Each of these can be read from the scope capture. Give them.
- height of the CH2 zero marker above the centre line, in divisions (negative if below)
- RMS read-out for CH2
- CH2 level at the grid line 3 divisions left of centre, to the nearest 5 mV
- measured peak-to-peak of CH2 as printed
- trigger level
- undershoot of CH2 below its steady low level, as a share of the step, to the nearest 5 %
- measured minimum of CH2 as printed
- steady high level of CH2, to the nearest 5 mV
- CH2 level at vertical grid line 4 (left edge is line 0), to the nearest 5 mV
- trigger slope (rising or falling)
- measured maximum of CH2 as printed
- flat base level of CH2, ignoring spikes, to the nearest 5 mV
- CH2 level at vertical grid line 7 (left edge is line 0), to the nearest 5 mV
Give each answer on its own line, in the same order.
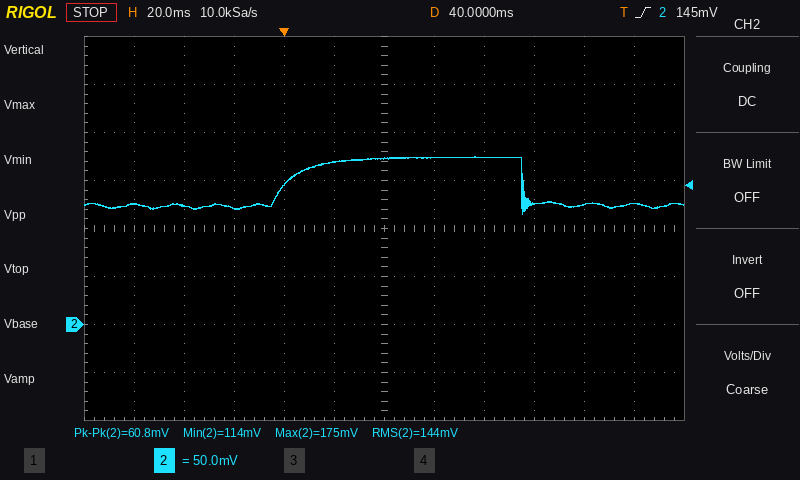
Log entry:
-2.0 div
144 mV
120 mV
60.8 mV
145 mV
20 %
114 mV
175 mV
145 mV
rising
175 mV
125 mV
175 mV
